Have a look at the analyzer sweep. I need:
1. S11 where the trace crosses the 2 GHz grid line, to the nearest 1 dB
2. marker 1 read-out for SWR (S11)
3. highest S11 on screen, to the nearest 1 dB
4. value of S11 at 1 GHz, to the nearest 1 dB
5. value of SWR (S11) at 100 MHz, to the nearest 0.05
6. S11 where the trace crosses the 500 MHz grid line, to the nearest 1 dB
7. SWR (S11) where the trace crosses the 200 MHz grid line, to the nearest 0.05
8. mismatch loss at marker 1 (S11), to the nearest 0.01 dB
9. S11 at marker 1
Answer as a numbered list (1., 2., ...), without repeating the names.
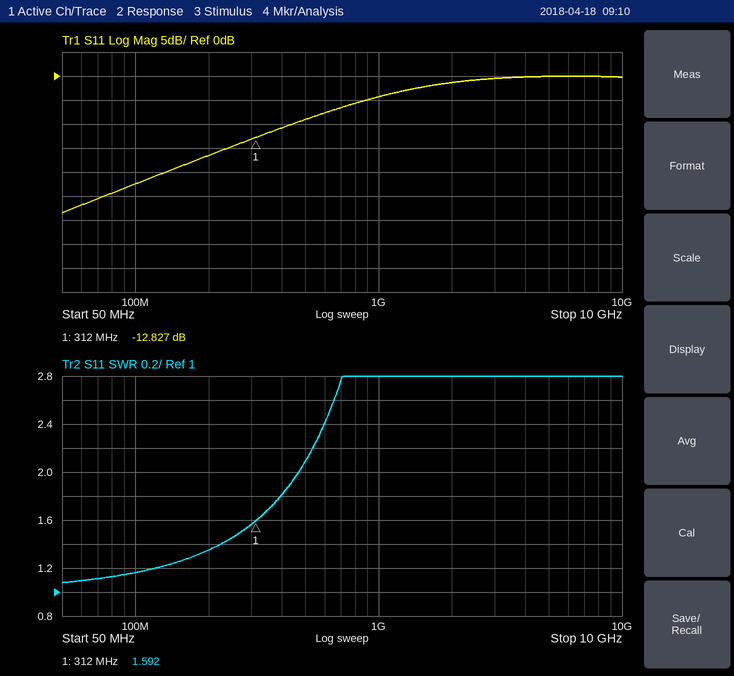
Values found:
1. -1 dB
2. 1.592
3. 0 dB
4. -4 dB
5. 1.15
6. -9 dB
7. 1.35
8. 0.23 dB
9. -12.827 dB
